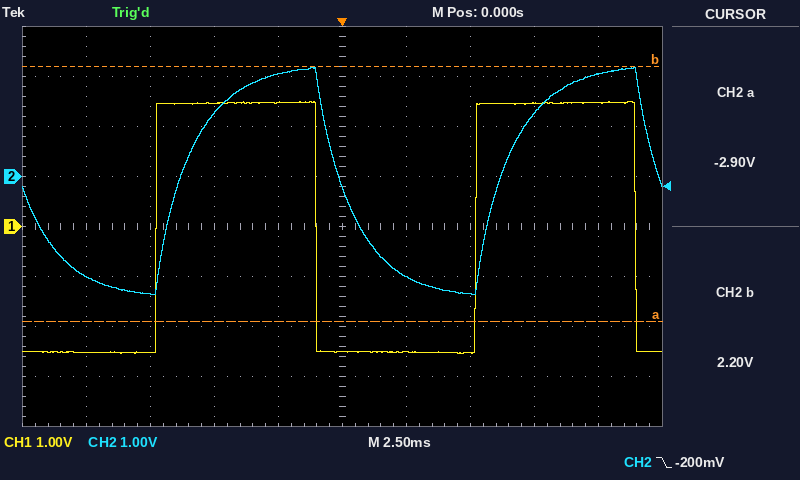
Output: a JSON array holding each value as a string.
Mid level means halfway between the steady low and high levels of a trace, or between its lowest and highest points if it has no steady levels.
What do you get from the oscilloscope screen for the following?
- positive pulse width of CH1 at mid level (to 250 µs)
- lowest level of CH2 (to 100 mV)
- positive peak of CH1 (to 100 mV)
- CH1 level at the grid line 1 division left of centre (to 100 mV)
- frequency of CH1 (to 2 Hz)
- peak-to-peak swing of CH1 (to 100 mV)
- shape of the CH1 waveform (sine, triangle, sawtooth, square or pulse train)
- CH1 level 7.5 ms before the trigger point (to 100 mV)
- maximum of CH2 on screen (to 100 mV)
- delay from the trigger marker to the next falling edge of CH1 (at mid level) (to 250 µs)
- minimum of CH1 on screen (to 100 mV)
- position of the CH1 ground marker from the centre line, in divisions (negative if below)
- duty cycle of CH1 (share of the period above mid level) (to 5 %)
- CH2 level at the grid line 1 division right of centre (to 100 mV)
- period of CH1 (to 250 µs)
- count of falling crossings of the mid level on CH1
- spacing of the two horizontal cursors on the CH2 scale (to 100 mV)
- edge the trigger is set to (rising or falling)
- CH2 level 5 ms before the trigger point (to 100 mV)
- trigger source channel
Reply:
["6.25 ms", "-2.4 V", "2.5 V", "2.5 V", "80 Hz", "5.0 V", "square", "-2.5 V", "2.2 V", "11.50 ms", "-2.5 V", "0.0 div", "50 %", "-2.0 V", "12.50 ms", "2", "5.1 V", "falling", "1.3 V", "CH2"]
